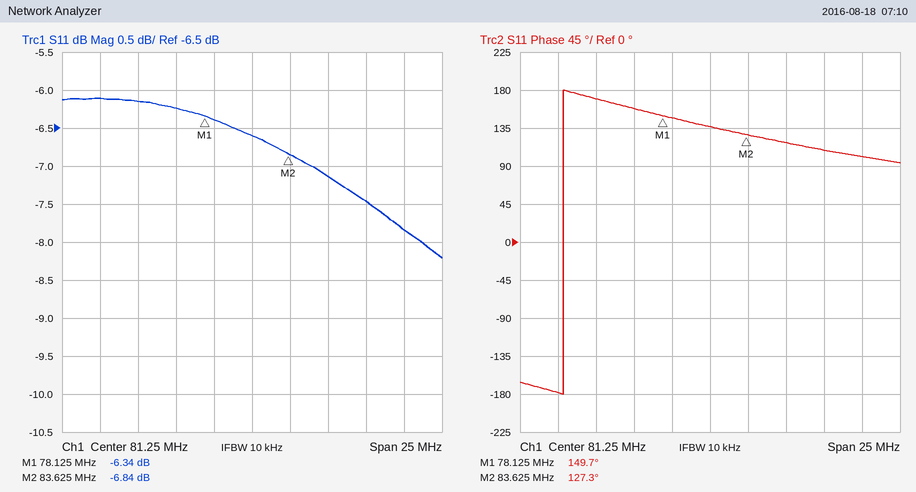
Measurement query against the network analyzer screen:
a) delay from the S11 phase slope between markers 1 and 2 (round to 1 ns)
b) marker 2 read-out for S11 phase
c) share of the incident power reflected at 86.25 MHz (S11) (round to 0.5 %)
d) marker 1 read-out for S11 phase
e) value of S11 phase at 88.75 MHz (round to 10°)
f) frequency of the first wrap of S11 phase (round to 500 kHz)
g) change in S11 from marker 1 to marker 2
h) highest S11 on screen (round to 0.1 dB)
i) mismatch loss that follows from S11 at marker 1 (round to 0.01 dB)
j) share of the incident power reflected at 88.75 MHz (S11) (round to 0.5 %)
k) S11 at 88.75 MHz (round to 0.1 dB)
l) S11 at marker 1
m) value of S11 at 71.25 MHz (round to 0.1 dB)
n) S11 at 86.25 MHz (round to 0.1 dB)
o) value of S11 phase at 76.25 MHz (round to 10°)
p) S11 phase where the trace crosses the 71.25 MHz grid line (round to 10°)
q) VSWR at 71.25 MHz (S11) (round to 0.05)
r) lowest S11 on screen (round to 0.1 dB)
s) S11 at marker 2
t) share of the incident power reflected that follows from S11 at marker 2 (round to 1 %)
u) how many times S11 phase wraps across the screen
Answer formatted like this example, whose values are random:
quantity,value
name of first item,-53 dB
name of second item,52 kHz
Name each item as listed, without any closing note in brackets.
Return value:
quantity,value
delay from the S11 phase slope between markers 1 and 2,11 ns
marker 2 read-out for S11 phase,127.3°
share of the incident power reflected at 86.25 MHz (S11),19.5 %
marker 1 read-out for S11 phase,149.7°
value of S11 phase at 88.75 MHz,110°
frequency of the first wrap of S11 phase,71.5 MHz
change in S11 from marker 1 to marker 2,-0.50 dB
highest S11 on screen,-6.1 dB
mismatch loss that follows from S11 at marker 1,1.15 dB
share of the incident power reflected at 88.75 MHz (S11),18.0 %
S11 at 88.75 MHz,-7.5 dB
S11 at marker 1,-6.34 dB
value of S11 at 71.25 MHz,-6.1 dB
S11 at 86.25 MHz,-7.1 dB
value of S11 phase at 76.25 MHz,160°
S11 phase where the trace crosses the 71.25 MHz grid line,-180°
VSWR at 71.25 MHz (S11),2.95
lowest S11 on screen,-8.2 dB
S11 at marker 2,-6.84 dB
share of the incident power reflected that follows from S11 at marker 2,21 %
how many times S11 phase wraps across the screen,1
